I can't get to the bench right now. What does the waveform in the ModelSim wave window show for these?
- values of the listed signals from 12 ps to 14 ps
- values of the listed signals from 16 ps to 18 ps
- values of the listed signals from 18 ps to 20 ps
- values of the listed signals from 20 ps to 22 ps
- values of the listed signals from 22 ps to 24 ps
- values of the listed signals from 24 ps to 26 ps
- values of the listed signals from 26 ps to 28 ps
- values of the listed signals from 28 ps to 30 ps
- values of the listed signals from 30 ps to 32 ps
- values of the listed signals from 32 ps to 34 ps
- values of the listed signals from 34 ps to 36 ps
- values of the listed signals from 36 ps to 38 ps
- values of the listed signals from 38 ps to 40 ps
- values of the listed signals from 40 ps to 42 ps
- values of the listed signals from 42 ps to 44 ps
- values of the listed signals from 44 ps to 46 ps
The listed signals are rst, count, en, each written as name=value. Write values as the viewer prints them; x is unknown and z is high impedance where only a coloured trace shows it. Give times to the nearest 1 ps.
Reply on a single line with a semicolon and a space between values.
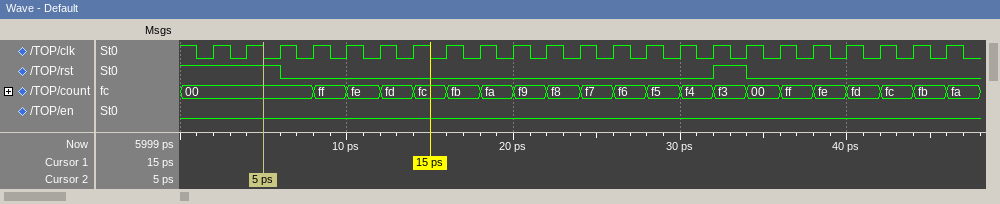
rst=0, count=fd, en=0; rst=0, count=fb, en=0; rst=0, count=fa, en=0; rst=0, count=f9, en=0; rst=0, count=f8, en=0; rst=0, count=f7, en=0; rst=0, count=f6, en=0; rst=0, count=f5, en=0; rst=0, count=f4, en=0; rst=1, count=f3, en=0; rst=0, count=00, en=0; rst=0, count=ff, en=0; rst=0, count=fe, en=0; rst=0, count=fd, en=0; rst=0, count=fc, en=0; rst=0, count=fb, en=0
